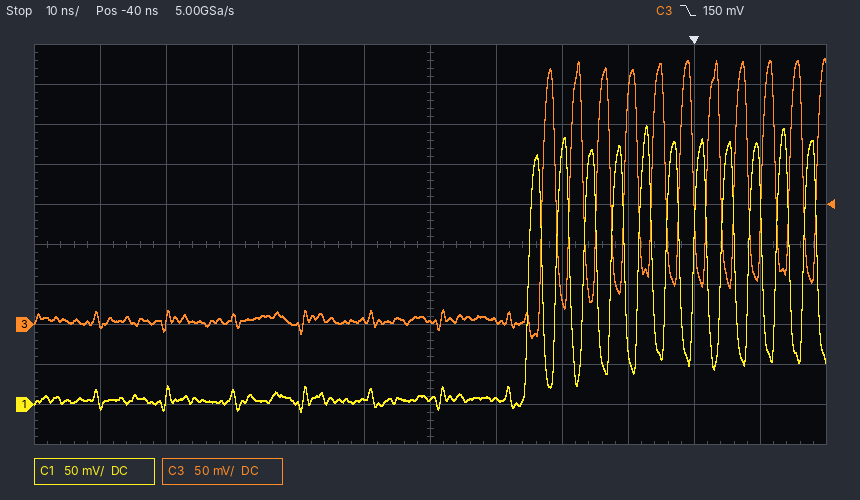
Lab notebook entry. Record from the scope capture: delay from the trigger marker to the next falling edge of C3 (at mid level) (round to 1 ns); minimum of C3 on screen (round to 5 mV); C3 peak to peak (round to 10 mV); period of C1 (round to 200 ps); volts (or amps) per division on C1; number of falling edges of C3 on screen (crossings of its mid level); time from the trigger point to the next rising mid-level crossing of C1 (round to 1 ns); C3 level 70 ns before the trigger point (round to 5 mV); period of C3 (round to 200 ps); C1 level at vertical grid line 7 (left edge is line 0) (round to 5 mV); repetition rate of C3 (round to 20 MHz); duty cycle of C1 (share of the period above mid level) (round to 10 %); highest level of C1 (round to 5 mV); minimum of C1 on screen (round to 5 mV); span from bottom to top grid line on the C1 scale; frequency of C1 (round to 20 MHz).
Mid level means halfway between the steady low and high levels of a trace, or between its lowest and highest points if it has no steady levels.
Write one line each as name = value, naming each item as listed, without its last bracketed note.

delay from the trigger marker to the next falling edge of C3 (at mid level) = 4 ns
minimum of C3 on screen = -15 mV
C3 peak to peak = 350 mV
period of C1 = 4.2 ns
volts (or amps) per division on C1 = 50 mV
number of falling edges of C3 on screen = 10
time from the trigger point to the next rising mid-level crossing of C1 = 4 ns
C3 level 70 ns before the trigger point = 10 mV
period of C3 = 4.2 ns
C1 level at vertical grid line 7 (left edge is line 0) = 5 mV
repetition rate of C3 = 240 MHz
duty cycle of C1 (share of the period above mid level) = 50 %
highest level of C1 = 350 mV
minimum of C1 on screen = -10 mV
span from bottom to top grid line on the C1 scale = 500 mV
frequency of C1 = 240 MHz
